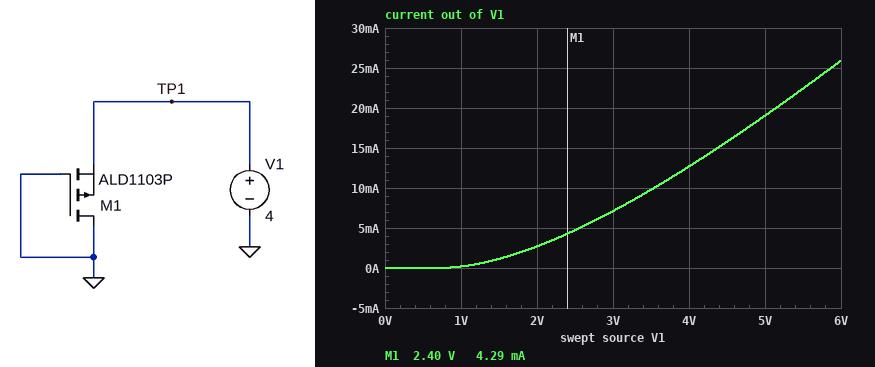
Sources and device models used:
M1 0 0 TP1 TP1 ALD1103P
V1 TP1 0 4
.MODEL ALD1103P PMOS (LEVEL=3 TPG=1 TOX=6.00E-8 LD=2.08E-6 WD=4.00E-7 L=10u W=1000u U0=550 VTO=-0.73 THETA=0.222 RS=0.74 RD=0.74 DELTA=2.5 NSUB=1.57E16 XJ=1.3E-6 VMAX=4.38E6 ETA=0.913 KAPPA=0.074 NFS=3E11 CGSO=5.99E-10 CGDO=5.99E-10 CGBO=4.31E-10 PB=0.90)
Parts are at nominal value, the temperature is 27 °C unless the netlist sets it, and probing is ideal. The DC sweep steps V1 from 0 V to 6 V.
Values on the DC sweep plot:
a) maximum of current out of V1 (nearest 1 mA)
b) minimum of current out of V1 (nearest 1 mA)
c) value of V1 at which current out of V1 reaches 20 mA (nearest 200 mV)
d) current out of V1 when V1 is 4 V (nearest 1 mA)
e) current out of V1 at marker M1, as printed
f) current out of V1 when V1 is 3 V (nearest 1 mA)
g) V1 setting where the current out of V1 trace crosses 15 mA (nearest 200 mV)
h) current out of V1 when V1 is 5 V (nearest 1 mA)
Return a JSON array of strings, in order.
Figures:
["26 mA", "0 A", "5.2 V", "13 mA", "4.29 mA", "7 mA", "4.4 V", "19 mA"]
